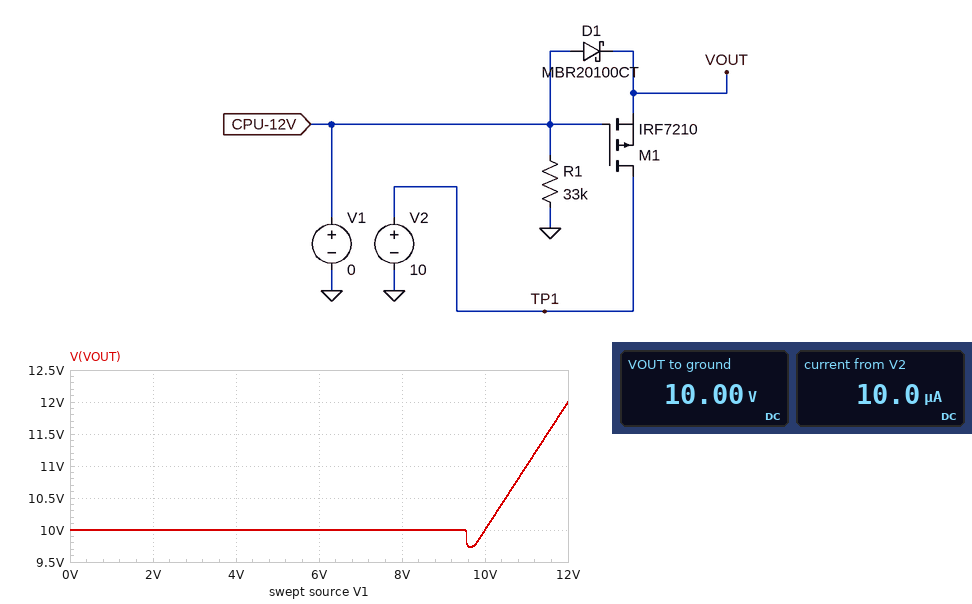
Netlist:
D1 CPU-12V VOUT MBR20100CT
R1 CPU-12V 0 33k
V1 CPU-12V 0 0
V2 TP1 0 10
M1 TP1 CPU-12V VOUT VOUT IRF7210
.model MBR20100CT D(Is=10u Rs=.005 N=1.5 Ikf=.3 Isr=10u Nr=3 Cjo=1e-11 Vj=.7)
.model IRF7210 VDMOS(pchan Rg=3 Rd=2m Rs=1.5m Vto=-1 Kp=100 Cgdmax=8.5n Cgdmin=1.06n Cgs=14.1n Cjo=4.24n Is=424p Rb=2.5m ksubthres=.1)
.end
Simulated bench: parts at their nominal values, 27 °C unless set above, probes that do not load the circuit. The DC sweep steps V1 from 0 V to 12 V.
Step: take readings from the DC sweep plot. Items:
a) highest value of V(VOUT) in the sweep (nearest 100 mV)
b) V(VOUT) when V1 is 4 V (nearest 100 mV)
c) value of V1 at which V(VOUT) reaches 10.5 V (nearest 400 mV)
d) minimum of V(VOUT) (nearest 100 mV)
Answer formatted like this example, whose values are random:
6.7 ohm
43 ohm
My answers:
12.0 V
10.0 V
10.4 V
9.7 V
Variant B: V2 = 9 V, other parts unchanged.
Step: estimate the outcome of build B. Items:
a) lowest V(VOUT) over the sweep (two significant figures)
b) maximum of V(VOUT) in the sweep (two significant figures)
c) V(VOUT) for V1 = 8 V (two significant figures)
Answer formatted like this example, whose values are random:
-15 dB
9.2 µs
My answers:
8.7 V
12 V
9.0 V
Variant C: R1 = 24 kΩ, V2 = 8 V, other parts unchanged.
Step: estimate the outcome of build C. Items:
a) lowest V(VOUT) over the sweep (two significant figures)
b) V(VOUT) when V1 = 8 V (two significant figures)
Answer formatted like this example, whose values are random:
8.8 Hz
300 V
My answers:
7.7 V
8.0 V
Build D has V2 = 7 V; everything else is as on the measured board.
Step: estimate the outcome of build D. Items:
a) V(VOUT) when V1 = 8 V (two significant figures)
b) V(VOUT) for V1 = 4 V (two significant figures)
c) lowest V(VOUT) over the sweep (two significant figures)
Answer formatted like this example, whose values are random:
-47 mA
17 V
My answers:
8.0 V
7.0 V
6.7 V
